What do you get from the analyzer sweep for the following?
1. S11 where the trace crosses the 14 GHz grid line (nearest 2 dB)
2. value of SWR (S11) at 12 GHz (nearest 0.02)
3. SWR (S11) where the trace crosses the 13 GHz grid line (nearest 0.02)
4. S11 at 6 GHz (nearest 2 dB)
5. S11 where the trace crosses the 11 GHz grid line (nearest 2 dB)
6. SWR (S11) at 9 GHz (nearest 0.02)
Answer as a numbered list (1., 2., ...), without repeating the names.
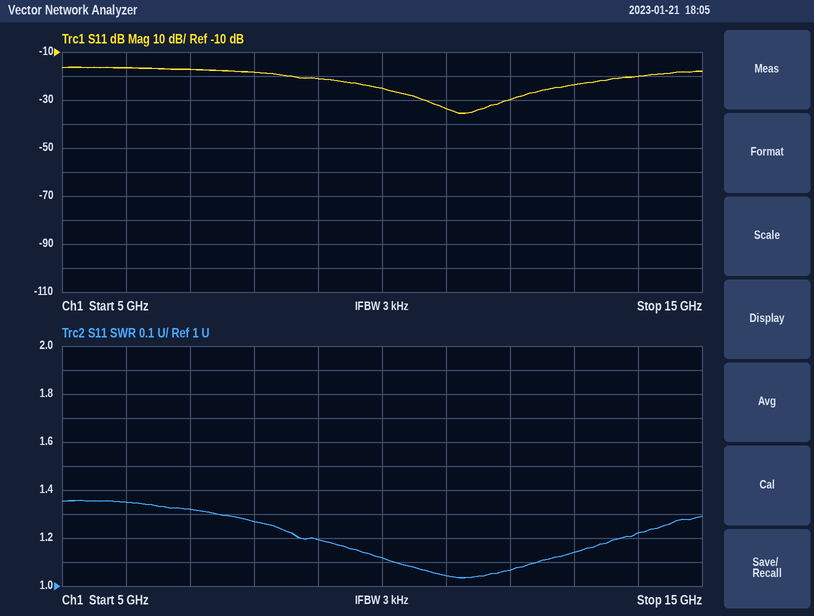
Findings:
1. -20 dB
2. 1.06
3. 1.14
4. -16 dB
5. -34 dB
6. 1.20
